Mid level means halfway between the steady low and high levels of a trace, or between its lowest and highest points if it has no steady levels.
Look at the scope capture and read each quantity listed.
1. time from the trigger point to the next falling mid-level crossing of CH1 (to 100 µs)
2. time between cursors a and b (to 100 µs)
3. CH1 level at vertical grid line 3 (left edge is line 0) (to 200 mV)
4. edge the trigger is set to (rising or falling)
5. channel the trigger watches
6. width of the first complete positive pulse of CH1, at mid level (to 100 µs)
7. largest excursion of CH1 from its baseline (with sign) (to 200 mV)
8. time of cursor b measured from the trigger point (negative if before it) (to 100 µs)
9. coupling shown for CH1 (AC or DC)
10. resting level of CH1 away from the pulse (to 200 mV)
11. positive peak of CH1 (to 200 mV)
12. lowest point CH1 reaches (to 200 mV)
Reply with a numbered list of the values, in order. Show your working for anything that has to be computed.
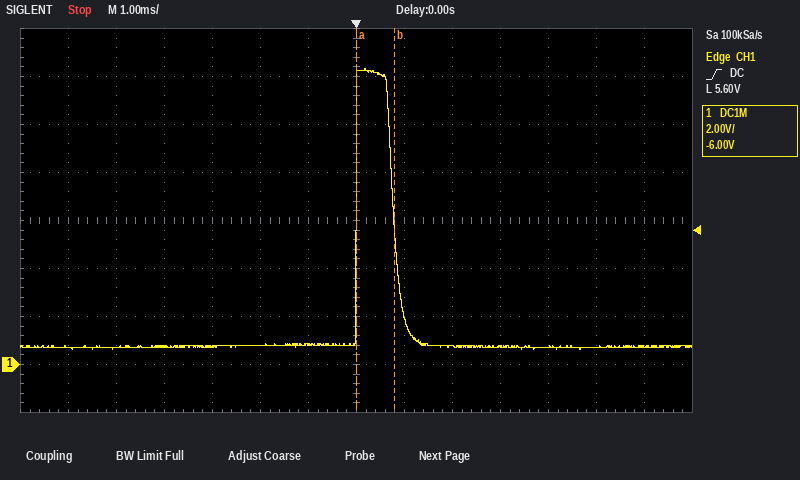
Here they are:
1. 800 µs
2. 800 µs
3. 800 mV
4. rising
5. CH1
6. 800 µs
7. 12.4 V − (800 mV) = +11.6 V
8. +800 µs
9. DC
10. 800 mV
11. 12.4 V
12. 600 mV
